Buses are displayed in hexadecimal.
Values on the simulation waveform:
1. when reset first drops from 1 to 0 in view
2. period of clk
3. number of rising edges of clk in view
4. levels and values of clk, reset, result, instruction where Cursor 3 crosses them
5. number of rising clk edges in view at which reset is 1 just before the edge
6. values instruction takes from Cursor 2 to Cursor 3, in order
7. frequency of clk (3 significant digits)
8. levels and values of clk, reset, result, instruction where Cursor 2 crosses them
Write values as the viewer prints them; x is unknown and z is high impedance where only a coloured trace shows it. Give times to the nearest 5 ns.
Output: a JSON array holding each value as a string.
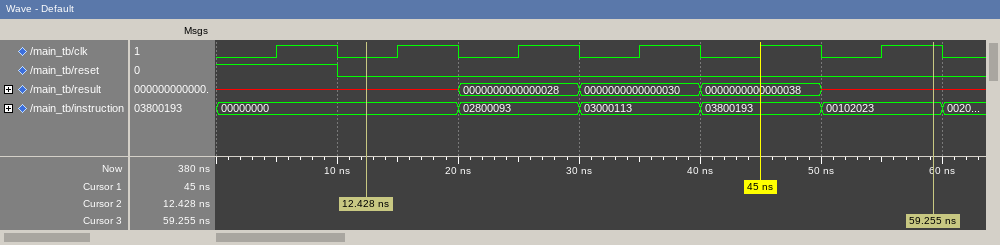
["10 ns", "10 ns", "6", "clk=1, reset=0, result=x, instruction=00102023", "1", "00000000, 02800093, 03000113, 03800193, 00102023", "100 MHz", "clk=0, reset=0, result=x, instruction=00000000"]
